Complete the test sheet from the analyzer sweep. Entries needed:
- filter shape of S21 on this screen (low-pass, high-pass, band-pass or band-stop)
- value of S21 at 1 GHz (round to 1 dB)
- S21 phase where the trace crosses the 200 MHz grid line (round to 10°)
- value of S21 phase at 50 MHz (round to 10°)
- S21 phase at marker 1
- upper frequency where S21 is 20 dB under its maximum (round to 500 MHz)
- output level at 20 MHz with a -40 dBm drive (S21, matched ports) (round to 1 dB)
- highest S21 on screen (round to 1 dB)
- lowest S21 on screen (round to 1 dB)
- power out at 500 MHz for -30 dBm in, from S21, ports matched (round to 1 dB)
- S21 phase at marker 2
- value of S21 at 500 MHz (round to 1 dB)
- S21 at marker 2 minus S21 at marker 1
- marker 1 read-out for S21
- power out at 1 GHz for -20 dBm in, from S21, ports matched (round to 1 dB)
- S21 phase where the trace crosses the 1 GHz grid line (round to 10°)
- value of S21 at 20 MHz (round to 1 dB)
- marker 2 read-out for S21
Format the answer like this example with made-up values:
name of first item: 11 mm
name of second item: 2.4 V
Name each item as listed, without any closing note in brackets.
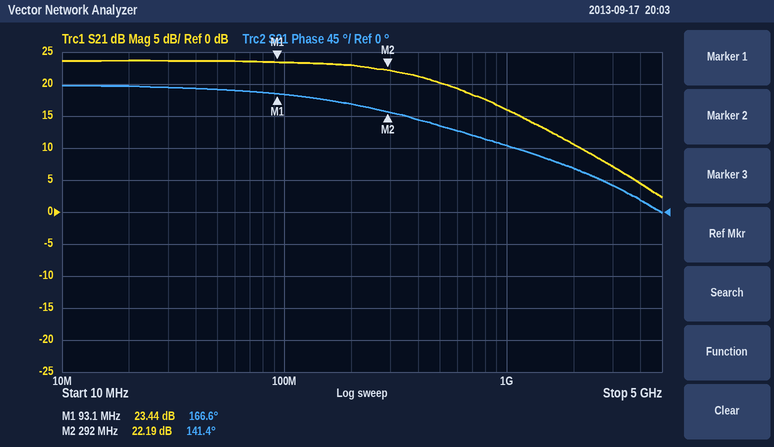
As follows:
filter shape of S21 on this screen: low-pass
value of S21 at 1 GHz: 16 dB
S21 phase where the trace crosses the 200 MHz grid line: 150°
value of S21 phase at 50 MHz: 170°
S21 phase at marker 1: 166.6°
upper frequency where S21 is 20 dB under its maximum: 4.5 GHz
output level at 20 MHz with a -40 dBm drive (S21, matched ports): -16 dBm
highest S21 on screen: 24 dB
lowest S21 on screen: 2 dB
power out at 500 MHz for -30 dBm in, from S21, ports matched: -10 dBm
S21 phase at marker 2: 141.4°
value of S21 at 500 MHz: 20 dB
S21 at marker 2 minus S21 at marker 1: -1.25 dB
marker 1 read-out for S21: 23.44 dB
power out at 1 GHz for -20 dBm in, from S21, ports matched: -4 dBm
S21 phase where the trace crosses the 1 GHz grid line: 90°
value of S21 at 20 MHz: 24 dB
marker 2 read-out for S21: 22.19 dB
